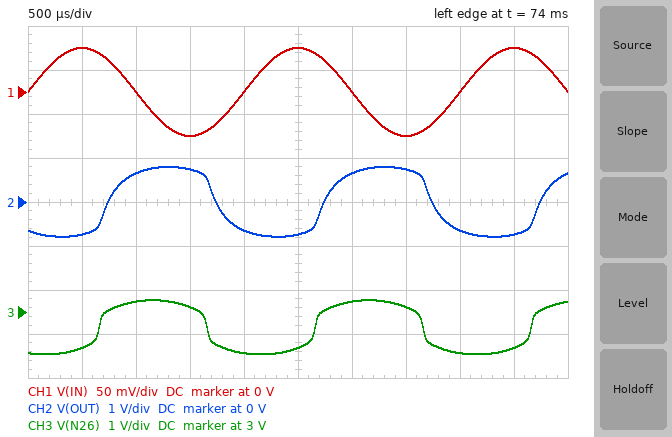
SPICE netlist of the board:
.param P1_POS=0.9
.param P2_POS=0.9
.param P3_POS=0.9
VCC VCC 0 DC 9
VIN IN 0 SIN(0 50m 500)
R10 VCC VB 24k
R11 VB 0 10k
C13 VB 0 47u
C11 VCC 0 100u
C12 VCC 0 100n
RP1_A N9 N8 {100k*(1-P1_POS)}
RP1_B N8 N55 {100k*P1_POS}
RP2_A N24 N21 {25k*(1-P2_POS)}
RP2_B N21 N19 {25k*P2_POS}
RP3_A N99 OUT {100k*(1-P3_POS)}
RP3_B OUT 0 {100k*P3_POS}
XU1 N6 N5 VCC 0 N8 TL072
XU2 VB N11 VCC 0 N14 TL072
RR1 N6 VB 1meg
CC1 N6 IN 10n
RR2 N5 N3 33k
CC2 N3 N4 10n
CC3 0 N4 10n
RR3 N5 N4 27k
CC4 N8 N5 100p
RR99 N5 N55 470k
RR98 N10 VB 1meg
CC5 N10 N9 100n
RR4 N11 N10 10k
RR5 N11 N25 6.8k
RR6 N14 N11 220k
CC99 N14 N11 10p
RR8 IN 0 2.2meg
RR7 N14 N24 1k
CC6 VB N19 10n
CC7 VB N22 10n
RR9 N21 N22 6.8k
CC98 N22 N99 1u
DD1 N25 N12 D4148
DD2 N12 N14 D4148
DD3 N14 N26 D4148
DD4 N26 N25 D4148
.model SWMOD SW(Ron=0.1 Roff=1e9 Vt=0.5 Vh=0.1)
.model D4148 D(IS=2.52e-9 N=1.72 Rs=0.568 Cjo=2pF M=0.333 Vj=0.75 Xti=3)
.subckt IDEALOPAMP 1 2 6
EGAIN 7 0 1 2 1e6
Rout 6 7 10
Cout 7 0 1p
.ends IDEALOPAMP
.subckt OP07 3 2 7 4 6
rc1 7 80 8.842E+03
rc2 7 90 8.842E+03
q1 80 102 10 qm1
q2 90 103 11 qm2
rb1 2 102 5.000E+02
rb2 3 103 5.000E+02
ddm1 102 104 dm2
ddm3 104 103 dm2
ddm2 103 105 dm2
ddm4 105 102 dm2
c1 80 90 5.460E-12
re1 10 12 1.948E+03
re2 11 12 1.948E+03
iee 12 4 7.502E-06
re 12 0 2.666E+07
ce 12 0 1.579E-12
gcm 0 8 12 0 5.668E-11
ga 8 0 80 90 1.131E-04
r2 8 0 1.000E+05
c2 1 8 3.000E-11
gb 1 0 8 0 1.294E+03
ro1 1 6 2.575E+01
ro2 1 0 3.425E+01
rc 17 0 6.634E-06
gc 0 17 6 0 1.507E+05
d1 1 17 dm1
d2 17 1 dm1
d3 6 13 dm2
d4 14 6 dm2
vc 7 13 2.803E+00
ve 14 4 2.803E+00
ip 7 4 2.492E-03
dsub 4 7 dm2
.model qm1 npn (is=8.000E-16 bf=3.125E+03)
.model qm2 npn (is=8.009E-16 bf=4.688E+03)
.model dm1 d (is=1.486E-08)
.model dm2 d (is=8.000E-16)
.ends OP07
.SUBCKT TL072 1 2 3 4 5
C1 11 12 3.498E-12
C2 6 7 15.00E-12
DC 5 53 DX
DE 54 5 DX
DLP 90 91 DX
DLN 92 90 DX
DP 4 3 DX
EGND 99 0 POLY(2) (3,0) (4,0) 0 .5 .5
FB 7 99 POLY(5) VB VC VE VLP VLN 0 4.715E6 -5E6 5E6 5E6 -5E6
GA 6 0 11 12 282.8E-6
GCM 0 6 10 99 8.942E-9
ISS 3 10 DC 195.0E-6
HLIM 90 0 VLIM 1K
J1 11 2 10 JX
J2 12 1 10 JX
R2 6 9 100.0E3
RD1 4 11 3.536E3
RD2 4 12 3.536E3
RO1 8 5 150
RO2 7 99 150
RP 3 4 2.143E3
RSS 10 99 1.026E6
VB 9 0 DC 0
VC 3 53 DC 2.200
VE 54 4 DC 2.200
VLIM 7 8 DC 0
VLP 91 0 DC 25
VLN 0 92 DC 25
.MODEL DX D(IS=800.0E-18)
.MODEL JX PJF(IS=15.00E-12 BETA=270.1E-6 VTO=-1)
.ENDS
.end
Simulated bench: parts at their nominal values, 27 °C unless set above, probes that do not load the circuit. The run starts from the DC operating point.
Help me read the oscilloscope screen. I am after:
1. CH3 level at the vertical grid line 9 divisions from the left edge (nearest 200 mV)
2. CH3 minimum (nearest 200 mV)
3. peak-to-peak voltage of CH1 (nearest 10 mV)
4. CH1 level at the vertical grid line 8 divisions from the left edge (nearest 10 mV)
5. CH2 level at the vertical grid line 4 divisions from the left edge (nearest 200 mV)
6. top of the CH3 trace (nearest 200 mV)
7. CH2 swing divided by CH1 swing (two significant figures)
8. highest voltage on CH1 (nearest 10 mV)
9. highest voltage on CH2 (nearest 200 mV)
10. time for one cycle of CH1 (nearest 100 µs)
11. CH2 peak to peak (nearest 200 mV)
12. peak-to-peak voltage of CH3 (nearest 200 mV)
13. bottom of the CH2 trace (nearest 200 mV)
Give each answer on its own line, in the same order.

2.2 V
2.0 V
100 mV
0 V
-600 mV
3.2 V
16
50 mV
800 mV
2.0 ms
1.6 V
1.2 V
-800 mV
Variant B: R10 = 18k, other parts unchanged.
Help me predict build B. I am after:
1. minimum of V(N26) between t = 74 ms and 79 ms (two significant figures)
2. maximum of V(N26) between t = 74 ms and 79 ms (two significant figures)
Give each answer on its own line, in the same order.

2.6 V
3.8 V
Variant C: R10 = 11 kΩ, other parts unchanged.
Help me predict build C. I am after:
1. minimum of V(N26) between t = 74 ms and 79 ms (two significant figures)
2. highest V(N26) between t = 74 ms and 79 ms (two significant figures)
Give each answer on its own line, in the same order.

3.7 V
4.9 V
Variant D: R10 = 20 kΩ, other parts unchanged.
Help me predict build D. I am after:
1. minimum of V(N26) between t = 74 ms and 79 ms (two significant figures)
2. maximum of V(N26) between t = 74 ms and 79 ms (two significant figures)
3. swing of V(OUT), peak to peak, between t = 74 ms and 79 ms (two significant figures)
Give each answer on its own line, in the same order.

2.4 V
3.6 V
1.6 V
